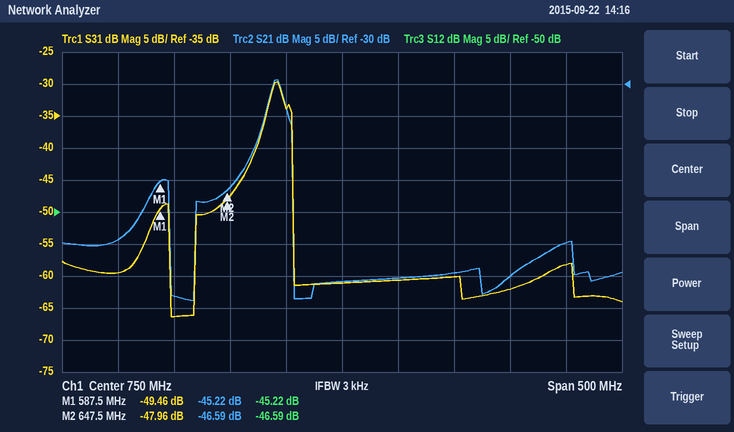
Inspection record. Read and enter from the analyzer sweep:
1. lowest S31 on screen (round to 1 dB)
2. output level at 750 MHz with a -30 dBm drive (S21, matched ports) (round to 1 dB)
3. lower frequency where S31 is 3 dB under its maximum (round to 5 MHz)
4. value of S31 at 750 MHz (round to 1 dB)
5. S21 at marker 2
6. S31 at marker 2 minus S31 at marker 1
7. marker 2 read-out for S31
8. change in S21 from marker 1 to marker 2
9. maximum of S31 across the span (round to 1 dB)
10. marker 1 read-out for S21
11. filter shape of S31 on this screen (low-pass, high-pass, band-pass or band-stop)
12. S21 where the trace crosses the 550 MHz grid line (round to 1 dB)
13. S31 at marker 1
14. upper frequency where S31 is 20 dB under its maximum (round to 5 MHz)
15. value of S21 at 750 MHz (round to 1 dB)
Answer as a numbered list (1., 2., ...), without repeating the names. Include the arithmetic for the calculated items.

1. -66 dB
2. -30 dBm + (-61 dB) = -91 dBm
3. 685 MHz
4. -61 dB
5. -46.59 dB
6. -47.96 − (-49.46) = 1.50 dB
7. -47.96 dB
8. -46.59 − (-45.22) = -1.37 dB
9. -30 dB
10. -45.22 dB
11. band-pass
12. -54 dB
13. -49.46 dB
14. 705 MHz
15. -61 dB
